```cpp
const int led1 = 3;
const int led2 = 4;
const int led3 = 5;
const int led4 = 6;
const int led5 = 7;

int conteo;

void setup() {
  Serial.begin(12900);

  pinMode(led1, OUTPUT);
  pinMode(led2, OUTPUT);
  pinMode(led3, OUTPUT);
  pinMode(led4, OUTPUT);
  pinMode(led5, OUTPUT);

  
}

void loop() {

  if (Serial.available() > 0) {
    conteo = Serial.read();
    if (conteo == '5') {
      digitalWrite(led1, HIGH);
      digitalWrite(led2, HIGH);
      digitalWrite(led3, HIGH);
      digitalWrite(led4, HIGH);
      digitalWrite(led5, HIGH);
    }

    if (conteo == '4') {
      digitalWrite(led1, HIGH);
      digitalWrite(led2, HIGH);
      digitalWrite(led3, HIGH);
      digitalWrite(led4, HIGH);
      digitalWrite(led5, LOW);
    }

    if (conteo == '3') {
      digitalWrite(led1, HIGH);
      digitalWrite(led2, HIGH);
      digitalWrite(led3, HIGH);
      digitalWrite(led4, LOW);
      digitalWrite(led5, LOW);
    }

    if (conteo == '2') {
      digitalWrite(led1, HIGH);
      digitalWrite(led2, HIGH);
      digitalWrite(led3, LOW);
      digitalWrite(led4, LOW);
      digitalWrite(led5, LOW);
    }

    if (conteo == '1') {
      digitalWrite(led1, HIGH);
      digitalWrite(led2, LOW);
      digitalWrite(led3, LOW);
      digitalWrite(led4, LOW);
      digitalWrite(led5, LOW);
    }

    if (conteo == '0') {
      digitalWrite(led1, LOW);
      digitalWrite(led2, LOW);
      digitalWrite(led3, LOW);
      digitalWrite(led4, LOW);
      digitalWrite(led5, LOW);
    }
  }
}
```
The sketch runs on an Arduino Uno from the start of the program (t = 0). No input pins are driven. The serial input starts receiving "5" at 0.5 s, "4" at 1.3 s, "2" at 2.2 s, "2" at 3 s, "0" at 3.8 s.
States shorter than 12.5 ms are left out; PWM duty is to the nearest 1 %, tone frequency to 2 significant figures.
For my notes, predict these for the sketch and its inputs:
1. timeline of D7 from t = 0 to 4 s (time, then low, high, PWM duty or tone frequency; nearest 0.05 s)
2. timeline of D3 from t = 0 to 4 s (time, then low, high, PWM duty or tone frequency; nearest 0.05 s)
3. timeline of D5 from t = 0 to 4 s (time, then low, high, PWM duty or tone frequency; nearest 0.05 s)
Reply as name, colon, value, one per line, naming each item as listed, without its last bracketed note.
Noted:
timeline of D7 from t = 0 to 4 s: 0 s low; 0.5 s high; 1.3 s low
timeline of D3 from t = 0 to 4 s: 0 s low; 0.5 s high; 3.8 s low
timeline of D5 from t = 0 to 4 s: 0 s low; 0.5 s high; 2.2 s low
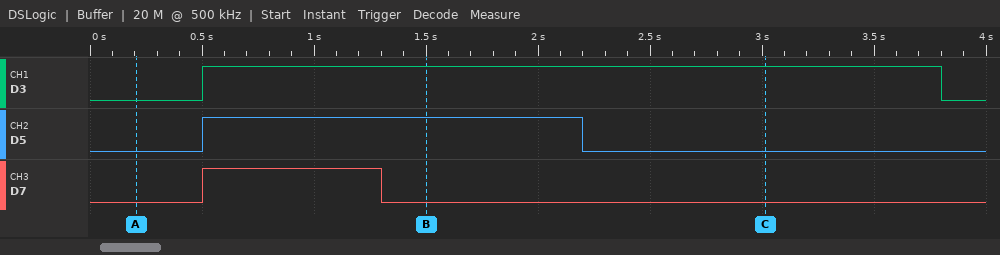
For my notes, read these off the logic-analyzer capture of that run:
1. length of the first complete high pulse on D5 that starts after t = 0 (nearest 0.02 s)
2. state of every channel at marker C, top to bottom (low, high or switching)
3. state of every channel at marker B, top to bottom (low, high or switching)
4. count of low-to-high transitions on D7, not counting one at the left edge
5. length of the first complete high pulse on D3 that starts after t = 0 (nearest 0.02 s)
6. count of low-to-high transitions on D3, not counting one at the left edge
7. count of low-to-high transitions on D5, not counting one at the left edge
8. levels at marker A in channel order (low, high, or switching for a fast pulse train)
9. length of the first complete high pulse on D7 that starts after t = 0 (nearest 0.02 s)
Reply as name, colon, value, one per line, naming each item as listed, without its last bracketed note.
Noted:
length of the first complete high pulse on D5 that starts after t = 0: 1.70 s
state of every channel at marker C, top to bottom: D3 high, D5 low, D7 low
state of every channel at marker B, top to bottom: D3 high, D5 high, D7 low
count of low-to-high transitions on D7, not counting one at the left edge: 1
length of the first complete high pulse on D3 that starts after t = 0: 3.30 s
count of low-to-high transitions on D3, not counting one at the left edge: 1
count of low-to-high transitions on D5, not counting one at the left edge: 1
levels at marker A in channel order: D3 low, D5 low, D7 low
length of the first complete high pulse on D7 that starts after t = 0: 0.80 s
